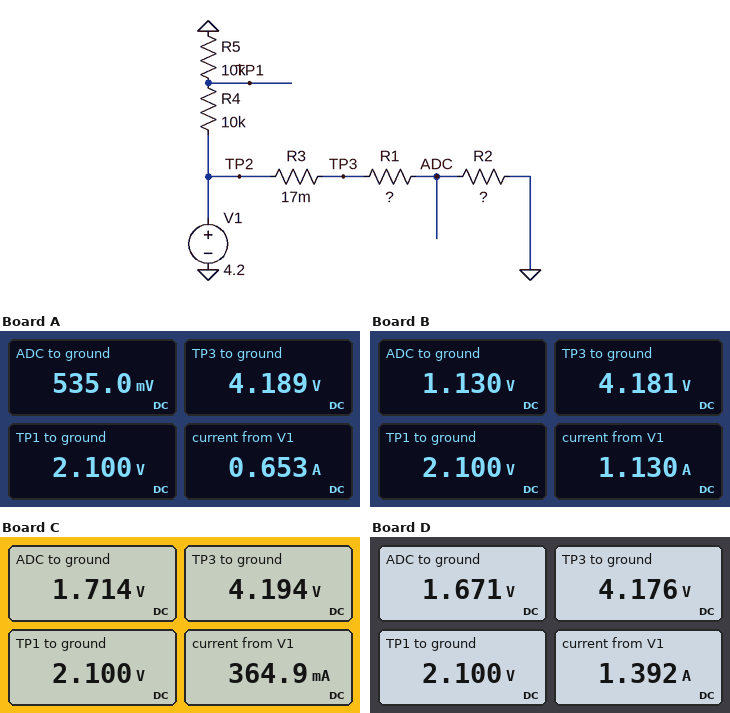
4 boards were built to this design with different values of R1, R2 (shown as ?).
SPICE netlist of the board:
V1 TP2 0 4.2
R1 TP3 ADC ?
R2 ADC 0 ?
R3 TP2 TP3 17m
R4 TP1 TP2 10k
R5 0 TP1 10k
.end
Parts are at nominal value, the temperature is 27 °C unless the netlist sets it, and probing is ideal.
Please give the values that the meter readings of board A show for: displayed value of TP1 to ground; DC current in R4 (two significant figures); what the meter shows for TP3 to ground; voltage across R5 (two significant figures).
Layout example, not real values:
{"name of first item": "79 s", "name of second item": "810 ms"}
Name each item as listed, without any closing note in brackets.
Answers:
{"displayed value of TP1 to ground": "2.100 V", "DC current in R4": "210 µA", "what the meter shows for TP3 to ground": "4.189 V", "voltage across R5": "2.1 V"}
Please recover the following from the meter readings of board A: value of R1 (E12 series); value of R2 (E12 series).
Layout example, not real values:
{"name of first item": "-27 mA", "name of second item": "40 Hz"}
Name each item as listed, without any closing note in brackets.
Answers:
{"value of R1": "5.6 Ω", "value of R2": "0.82 Ω"}
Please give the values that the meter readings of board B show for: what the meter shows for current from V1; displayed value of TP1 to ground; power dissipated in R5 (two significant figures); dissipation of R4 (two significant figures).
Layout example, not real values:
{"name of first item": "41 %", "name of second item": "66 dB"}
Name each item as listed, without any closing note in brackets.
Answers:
{"what the meter shows for current from V1": "1.130 A", "displayed value of TP1 to ground": "2.100 V", "power dissipated in R5": "440 µW", "dissipation of R4": "440 µW"}
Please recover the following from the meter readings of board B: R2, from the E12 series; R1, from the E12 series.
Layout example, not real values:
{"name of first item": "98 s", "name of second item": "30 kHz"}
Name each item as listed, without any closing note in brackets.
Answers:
{"R2, from the E12 series": "1 Ω", "R1, from the E12 series": "2.7 Ω"}
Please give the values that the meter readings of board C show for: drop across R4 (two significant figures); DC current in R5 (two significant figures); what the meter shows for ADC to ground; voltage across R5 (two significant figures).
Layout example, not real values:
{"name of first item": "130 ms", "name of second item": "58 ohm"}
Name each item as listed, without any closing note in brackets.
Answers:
{"drop across R4": "2.1 V", "DC current in R5": "210 µA", "what the meter shows for ADC to ground": "1.714 V", "voltage across R5": "2.1 V"}
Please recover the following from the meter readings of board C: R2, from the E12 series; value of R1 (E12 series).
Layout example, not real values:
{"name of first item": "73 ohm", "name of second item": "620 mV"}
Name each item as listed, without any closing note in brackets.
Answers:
{"R2, from the E12 series": "4.7 Ω", "value of R1": "6.8 Ω"}
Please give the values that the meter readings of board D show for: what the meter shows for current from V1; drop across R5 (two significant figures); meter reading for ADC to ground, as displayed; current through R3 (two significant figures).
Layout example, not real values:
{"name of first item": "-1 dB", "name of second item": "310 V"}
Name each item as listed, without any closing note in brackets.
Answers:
{"what the meter shows for current from V1": "1.392 A", "drop across R5": "2.1 V", "meter reading for ADC to ground, as displayed": "1.671 V", "current through R3": "1.4 A"}
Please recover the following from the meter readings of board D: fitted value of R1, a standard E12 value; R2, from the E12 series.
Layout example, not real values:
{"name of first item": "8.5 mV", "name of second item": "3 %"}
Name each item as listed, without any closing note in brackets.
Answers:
{"fitted value of R1, a standard E12 value": "1.8 Ω", "R2, from the E12 series": "1.2 Ω"}
